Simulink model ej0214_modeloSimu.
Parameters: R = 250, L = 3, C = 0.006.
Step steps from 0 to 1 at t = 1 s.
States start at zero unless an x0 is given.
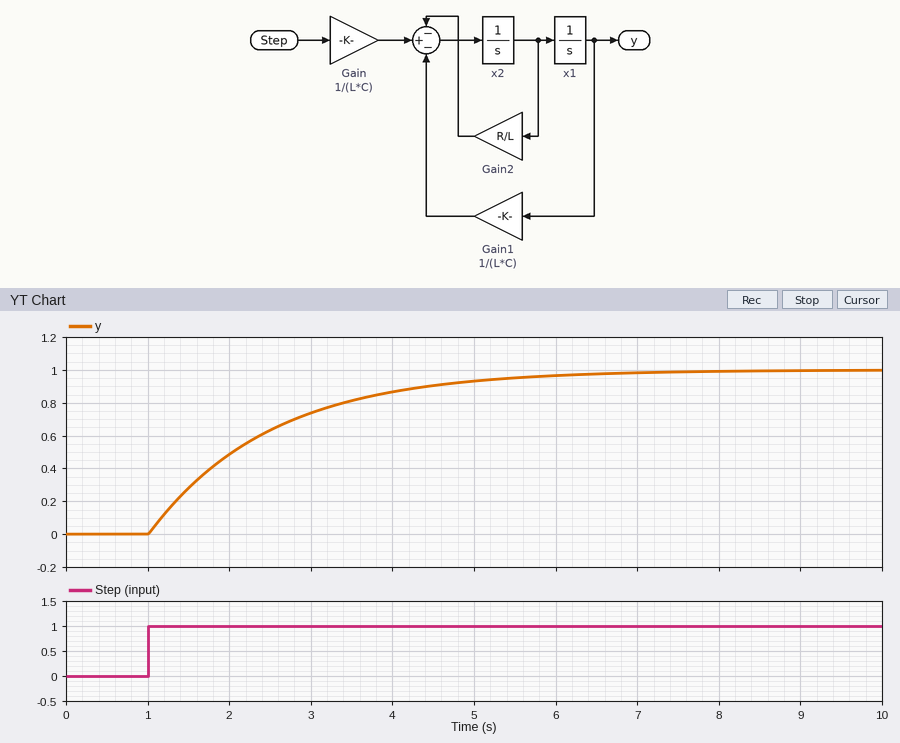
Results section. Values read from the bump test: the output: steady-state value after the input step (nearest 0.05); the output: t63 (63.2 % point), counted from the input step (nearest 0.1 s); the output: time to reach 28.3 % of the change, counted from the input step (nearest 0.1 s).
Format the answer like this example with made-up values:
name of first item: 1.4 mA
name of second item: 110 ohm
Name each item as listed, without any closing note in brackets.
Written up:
the output: steady-state value after the input step: 1.00
the output: t63 (63.2 % point), counted from the input step: 1.5 s
the output: time to reach 28.3 % of the change, counted from the input step: 0.5 s
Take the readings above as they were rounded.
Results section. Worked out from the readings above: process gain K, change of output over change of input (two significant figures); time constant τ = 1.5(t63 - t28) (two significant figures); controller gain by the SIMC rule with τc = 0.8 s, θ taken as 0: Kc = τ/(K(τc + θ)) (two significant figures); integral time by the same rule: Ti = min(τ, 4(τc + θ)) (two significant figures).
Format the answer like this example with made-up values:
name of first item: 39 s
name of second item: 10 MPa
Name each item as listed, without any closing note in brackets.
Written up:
process gain K, change of output over change of input: 1.0
time constant τ = 1.5(t63 - t28): 1.5 s
controller gain by the SIMC rule with τc = 0.8 s, θ taken as 0: Kc = τ/(K(τc + θ)): 1.9
integral time by the same rule: Ti = min(τ, 4(τc + θ)): 1.5 s
